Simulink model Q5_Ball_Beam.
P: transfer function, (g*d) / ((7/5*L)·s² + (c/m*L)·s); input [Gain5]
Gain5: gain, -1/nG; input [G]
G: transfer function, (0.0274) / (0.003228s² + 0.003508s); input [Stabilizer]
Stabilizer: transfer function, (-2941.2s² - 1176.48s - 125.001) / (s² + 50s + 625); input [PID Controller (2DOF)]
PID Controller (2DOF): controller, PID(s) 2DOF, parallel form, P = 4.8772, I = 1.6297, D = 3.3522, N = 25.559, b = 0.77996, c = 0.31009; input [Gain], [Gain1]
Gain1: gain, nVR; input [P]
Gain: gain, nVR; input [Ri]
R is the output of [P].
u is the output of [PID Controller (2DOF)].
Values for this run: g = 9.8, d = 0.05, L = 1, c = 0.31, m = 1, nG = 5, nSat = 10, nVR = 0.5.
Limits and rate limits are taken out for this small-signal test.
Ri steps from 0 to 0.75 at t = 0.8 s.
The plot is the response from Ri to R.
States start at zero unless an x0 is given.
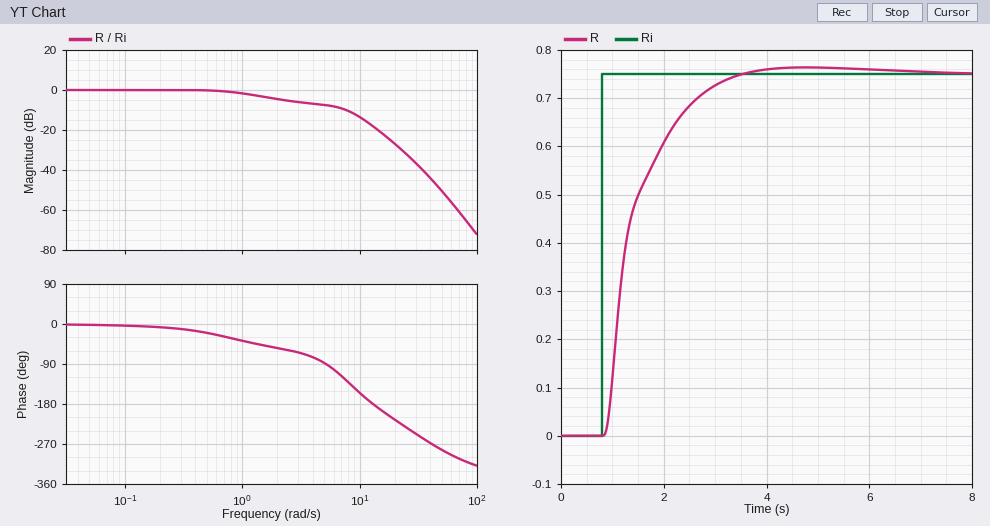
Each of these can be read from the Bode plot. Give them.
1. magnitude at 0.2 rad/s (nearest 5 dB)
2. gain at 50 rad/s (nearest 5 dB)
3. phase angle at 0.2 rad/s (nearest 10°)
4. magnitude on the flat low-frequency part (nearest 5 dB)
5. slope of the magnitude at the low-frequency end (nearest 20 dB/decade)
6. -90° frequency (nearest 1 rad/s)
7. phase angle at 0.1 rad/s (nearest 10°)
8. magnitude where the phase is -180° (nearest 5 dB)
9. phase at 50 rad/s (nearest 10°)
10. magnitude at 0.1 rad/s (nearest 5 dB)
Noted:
0 dB
-50 dB
-10°
0 dB
0 dB/decade
5 rad/s
0°
-20 dB
-280°
0 dB
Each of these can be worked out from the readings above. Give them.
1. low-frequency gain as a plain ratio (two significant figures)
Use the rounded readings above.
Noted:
1.0
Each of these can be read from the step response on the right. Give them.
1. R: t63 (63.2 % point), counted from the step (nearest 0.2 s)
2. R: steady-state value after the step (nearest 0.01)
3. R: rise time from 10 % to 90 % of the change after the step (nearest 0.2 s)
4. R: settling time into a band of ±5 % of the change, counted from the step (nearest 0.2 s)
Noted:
0.6 s
0.75
1.4 s
2.0 s
